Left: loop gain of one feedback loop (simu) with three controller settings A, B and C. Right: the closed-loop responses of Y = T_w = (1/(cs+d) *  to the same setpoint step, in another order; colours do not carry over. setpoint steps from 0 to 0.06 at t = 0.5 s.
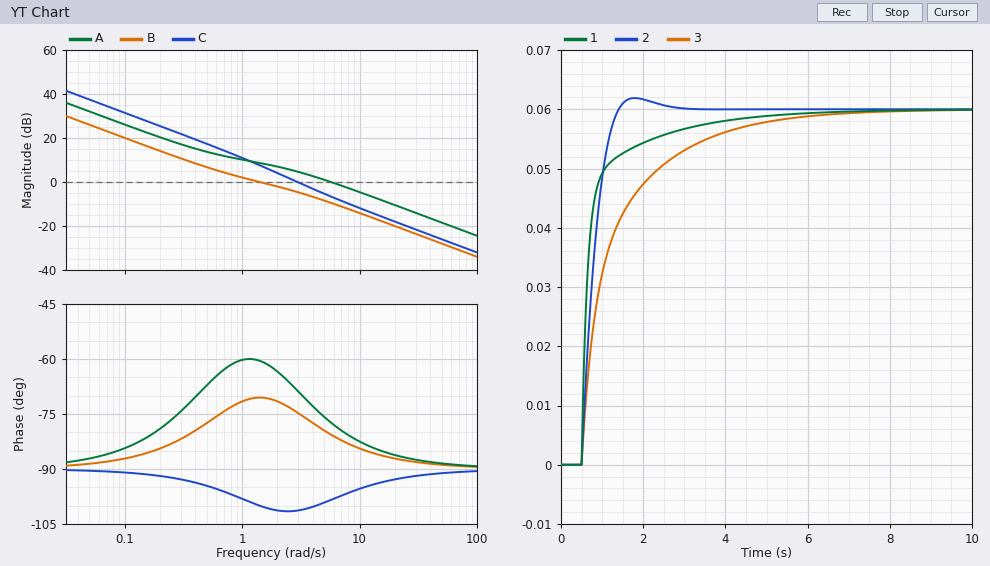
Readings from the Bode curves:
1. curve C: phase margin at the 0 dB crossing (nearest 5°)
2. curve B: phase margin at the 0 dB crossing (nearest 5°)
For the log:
80°
110°
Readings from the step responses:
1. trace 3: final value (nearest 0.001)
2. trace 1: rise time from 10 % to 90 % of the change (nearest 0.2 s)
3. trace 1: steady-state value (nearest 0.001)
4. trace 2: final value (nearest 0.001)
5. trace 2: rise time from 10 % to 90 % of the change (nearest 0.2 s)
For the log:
0.060
1.4 s
0.060
0.060
0.6 s
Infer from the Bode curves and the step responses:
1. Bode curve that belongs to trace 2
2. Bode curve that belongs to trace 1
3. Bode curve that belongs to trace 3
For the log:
C
A
B
